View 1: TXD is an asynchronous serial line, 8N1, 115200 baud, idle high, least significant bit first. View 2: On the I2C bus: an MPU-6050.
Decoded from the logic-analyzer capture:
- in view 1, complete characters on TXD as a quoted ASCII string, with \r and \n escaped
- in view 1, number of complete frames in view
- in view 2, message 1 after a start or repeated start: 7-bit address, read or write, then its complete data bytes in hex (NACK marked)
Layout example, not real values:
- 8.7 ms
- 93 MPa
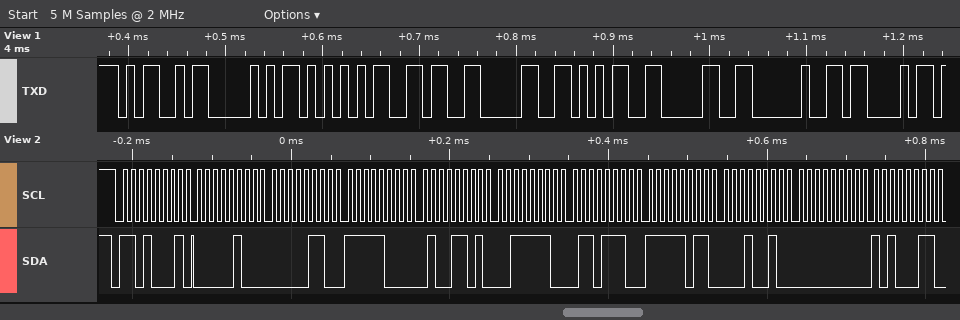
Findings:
- "MPU6050 C"
- 9
- 0x68 read: 04 06 F8 4D 3E 6E FB 12 00 A3
